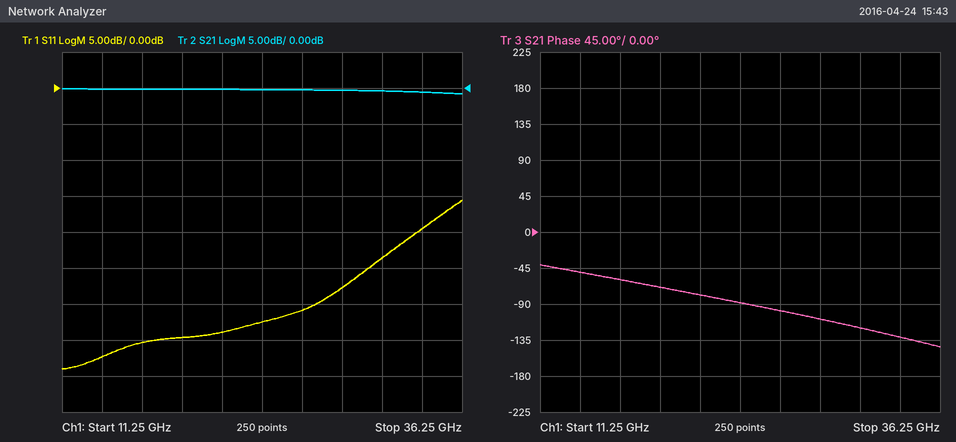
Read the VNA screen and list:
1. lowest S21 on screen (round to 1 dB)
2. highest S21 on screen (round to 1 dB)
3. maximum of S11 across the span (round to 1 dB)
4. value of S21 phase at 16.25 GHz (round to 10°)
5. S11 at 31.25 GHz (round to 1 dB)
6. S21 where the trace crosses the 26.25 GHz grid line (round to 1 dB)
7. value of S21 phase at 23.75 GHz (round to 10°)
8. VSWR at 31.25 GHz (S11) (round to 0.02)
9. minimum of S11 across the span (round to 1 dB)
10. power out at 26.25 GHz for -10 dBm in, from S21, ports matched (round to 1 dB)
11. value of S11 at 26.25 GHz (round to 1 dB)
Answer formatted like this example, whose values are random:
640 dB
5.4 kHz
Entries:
-1 dB
0 dB
-16 dB
-60°
-24 dB
0 dB
-90°
1.14
-39 dB
-10 dBm
-31 dB
